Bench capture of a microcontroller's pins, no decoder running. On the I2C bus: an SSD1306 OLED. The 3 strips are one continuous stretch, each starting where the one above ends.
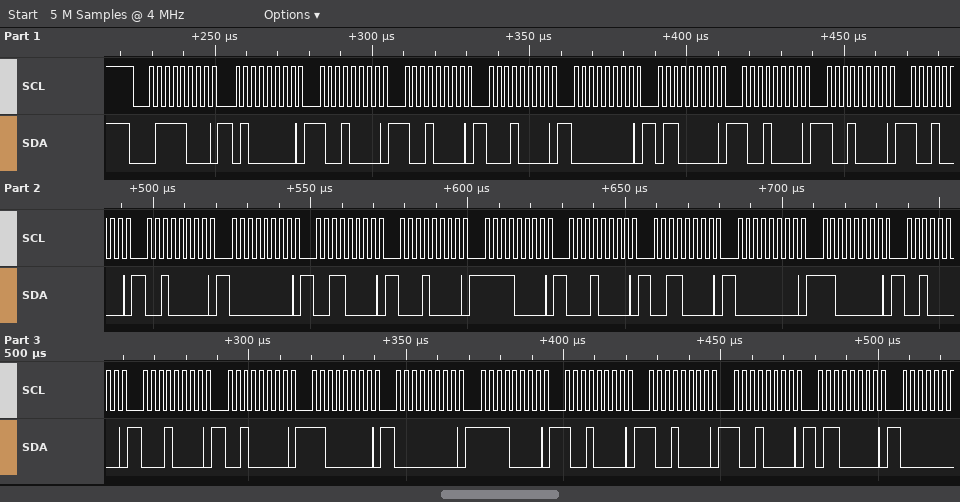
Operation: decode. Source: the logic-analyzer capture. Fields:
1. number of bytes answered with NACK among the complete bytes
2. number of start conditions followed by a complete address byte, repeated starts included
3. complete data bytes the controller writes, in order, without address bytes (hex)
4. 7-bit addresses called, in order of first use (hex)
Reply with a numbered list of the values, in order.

1. 0
2. 1
3. 40 90 90 10 00 60 90 90 90 20 00 30 10 F0 10 30 00 C0 20 10 20 C0 00 F0 90 90 90 60
4. 0x3C
